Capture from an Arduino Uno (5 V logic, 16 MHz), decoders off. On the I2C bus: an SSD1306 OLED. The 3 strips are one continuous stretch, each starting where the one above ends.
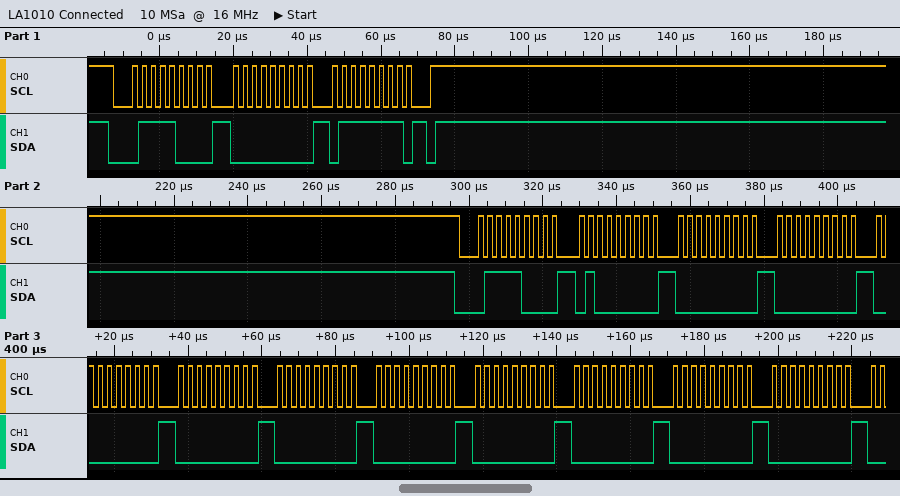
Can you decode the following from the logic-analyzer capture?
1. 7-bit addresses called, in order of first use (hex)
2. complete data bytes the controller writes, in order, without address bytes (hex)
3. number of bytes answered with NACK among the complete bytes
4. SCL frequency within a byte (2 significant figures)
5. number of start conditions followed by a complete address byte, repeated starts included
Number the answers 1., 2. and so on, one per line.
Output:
1. 0x3C
2. 00 7F 40 00 00 00 00 00 00 00 00 00 00
3. 0
4. 400 kHz
5. 2
